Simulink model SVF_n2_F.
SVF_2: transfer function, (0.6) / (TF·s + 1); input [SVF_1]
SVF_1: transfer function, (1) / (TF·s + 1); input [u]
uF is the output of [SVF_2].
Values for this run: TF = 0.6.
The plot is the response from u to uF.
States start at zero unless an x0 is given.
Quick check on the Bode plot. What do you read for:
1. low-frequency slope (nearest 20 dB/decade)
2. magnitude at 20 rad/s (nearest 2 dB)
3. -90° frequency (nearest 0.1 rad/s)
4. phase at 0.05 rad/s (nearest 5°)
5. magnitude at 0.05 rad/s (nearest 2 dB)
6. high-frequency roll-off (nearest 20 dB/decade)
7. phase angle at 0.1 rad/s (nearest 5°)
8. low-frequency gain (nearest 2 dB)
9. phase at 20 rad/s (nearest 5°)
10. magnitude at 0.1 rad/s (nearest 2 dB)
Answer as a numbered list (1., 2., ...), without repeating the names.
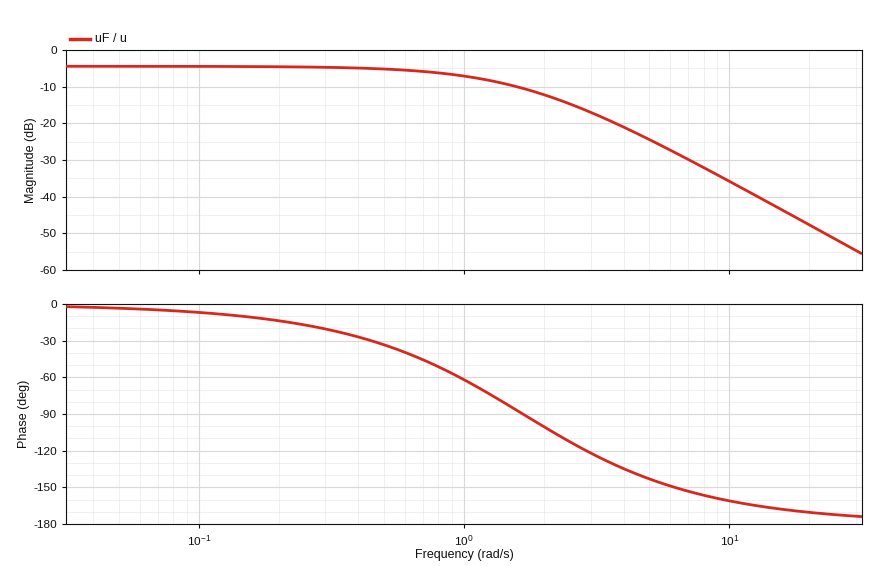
1. 0 dB/decade
2. -48 dB
3. 1.7 rad/s
4. -5°
5. -4 dB
6. -40 dB/decade
7. -5°
8. -4 dB
9. -170°
10. -4 dB
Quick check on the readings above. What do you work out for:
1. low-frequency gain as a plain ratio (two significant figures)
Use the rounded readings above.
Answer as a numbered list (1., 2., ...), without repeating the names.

1. 0.63
